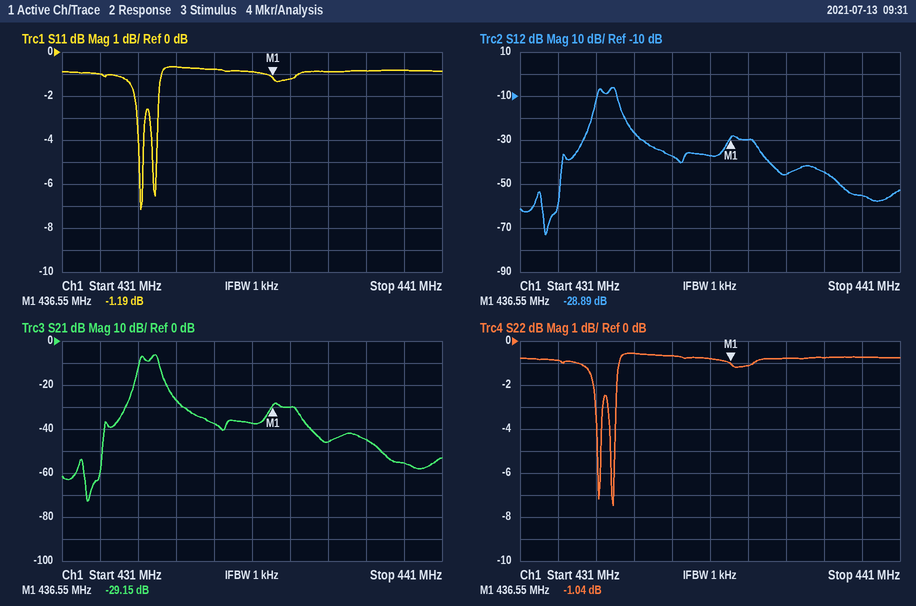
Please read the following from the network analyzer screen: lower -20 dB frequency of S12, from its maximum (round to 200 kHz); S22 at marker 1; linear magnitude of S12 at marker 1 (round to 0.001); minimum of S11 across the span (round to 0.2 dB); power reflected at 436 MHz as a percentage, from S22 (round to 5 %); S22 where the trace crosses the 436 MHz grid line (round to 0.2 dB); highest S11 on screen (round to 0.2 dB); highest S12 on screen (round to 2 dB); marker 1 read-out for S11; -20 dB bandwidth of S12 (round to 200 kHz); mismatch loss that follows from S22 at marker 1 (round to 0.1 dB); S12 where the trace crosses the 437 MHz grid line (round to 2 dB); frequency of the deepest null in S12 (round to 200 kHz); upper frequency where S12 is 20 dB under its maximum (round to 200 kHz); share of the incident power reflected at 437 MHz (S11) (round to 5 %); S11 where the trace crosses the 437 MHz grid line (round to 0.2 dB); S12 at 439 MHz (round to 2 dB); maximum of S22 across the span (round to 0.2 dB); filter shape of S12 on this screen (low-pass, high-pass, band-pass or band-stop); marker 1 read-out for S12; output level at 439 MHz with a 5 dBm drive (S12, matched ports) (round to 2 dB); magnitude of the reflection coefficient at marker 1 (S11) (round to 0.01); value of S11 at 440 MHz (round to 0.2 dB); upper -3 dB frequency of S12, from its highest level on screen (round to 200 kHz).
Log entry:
432.8 MHz
-1.04 dB
0.036
-7.2 dB
85 %
-0.8 dB
-0.6 dB
-6 dB
-1.19 dB
1.2 MHz
6.7 dB
-30 dB
431.6 MHz
434.0 MHz
75 %
-1.2 dB
-44 dB
-0.6 dB
band-pass
-28.89 dB
-40 dBm
0.87
-0.8 dB
433.6 MHz
